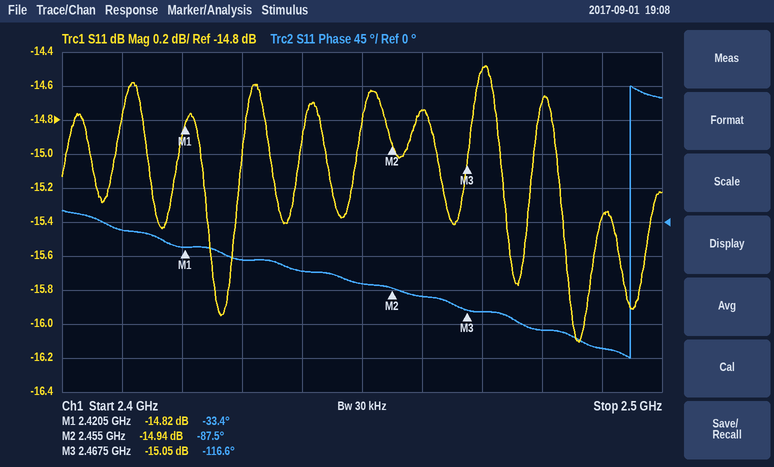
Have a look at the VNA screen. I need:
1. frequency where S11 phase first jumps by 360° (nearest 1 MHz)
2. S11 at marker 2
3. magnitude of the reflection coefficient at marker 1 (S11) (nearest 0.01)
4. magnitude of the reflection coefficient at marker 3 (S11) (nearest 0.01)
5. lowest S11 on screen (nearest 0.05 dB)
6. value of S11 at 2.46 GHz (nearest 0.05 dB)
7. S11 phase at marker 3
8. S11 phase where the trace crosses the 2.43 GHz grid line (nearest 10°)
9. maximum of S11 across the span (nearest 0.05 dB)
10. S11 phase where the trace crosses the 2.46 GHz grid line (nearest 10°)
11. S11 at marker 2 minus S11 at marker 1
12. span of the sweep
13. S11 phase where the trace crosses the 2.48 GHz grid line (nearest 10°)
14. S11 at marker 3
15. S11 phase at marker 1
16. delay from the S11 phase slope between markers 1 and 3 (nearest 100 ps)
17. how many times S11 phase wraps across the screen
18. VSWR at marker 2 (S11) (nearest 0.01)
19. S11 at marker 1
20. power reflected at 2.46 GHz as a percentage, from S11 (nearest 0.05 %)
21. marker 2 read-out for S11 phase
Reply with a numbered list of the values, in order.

1. 2.495 GHz
2. -14.94 dB
3. 0.18
4. 0.18
5. -16.10 dB
6. -14.75 dB
7. -116.6°
8. -50°
9. -14.50 dB
10. -100°
11. -0.12 dB
12. 100 MHz
13. -140°
14. -15.05 dB
15. -33.4°
16. 4.9 ns
17. 1
18. 1.44
19. -14.82 dB
20. 3.35 %
21. -87.5°
